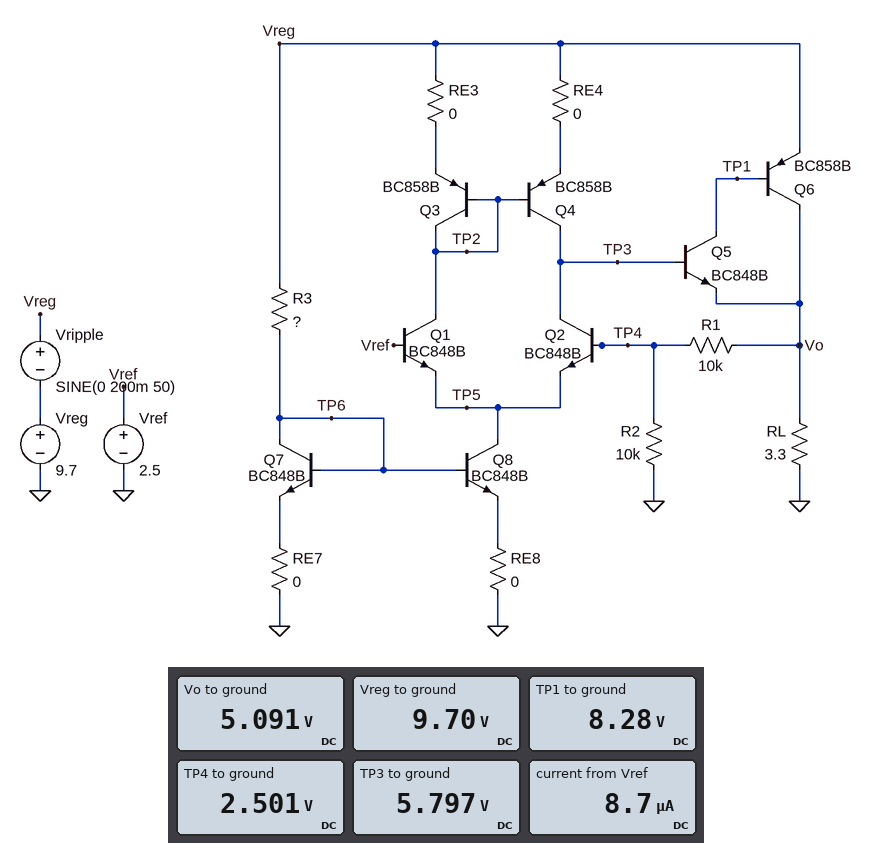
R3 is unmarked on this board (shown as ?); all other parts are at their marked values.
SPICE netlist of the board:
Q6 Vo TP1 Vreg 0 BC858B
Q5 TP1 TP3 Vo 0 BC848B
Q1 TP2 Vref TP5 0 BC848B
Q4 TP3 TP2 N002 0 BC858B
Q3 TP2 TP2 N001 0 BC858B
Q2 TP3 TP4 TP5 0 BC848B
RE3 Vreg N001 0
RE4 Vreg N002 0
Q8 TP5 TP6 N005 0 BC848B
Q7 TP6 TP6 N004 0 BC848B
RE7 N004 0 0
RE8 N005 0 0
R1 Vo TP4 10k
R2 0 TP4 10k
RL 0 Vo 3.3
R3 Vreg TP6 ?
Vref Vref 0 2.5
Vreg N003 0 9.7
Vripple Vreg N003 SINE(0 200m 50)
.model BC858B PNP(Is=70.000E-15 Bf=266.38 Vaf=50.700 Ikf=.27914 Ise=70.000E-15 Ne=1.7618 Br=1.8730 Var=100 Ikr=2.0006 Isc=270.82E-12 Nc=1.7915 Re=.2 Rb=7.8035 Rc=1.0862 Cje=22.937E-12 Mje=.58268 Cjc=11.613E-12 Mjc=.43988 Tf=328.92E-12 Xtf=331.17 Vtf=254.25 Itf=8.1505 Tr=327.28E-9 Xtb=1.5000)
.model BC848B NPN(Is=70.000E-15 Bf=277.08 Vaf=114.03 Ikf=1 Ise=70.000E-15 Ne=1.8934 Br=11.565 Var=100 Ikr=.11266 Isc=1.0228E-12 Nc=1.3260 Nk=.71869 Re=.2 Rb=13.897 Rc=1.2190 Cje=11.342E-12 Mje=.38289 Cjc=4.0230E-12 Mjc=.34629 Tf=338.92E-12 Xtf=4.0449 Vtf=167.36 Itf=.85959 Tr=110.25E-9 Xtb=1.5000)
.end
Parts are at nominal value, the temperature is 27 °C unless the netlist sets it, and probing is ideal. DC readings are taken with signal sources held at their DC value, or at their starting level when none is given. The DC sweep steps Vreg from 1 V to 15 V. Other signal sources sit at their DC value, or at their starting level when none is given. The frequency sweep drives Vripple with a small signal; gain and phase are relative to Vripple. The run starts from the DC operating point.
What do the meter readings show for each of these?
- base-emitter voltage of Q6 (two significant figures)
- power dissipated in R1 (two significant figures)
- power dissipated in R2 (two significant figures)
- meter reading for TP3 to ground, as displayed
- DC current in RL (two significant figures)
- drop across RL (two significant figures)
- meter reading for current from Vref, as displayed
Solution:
-1.4 V
670 µW
630 µW
5.797 V
1.5 A
5.1 V
8.7 µA
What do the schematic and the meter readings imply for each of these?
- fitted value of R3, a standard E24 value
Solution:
1.8 kΩ
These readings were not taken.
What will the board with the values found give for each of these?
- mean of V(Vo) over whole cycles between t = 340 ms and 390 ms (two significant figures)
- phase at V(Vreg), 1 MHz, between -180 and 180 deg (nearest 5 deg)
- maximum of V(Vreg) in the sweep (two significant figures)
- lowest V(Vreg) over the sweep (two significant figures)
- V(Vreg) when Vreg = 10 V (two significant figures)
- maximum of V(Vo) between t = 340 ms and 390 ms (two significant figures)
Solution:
5.1 V
0 deg
15 V
1.0 V
10 V
5.1 V
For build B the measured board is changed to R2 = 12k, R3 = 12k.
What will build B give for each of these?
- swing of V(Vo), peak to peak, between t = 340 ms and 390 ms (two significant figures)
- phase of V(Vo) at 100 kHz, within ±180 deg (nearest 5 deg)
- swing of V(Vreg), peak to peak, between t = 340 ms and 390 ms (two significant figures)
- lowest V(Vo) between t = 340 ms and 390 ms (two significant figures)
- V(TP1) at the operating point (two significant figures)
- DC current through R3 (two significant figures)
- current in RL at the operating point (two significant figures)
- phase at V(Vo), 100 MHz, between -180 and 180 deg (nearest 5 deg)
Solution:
2.0 mV
25 deg
400 mV
4.6 V
8.4 V
760 µA
1.4 A
5 deg
